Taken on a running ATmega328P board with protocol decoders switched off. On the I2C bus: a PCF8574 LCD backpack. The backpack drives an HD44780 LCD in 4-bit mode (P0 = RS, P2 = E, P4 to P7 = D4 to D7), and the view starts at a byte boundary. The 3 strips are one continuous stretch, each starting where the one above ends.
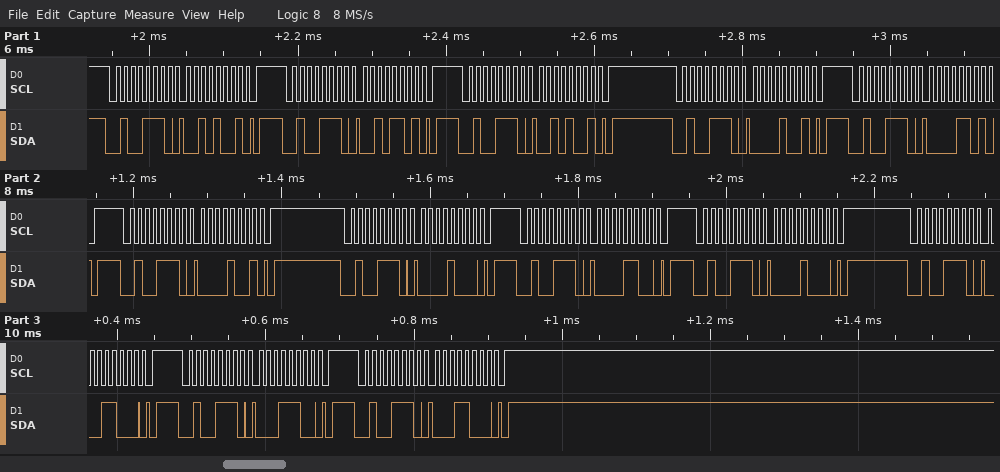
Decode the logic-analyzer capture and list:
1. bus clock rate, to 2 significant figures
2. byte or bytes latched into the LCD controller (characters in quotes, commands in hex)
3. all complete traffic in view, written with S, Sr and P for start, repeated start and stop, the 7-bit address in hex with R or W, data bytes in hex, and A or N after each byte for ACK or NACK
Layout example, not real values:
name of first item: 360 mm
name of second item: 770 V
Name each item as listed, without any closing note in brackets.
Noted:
bus clock rate, to 2 significant figures: 100 kHz
byte or bytes latched into the LCD controller: ' ' 0x01
all complete traffic in view, written with S, Sr and P for start, repeated start and stop, the 7-bit address in hex with R or W, data bytes in hex, and A or N after each byte for ACK or NACK: S 27W A 29 A P S 27W A 2D A P S 27W A 29 A P S 27W A 09 A P S 27W A 0D A P S 27W A 09 A P S 27W A 08 A P S 27W A 0C A P S 27W A 08 A P S 27W A 18 A P S 27W A 1C A P S 27W A 18 A P
